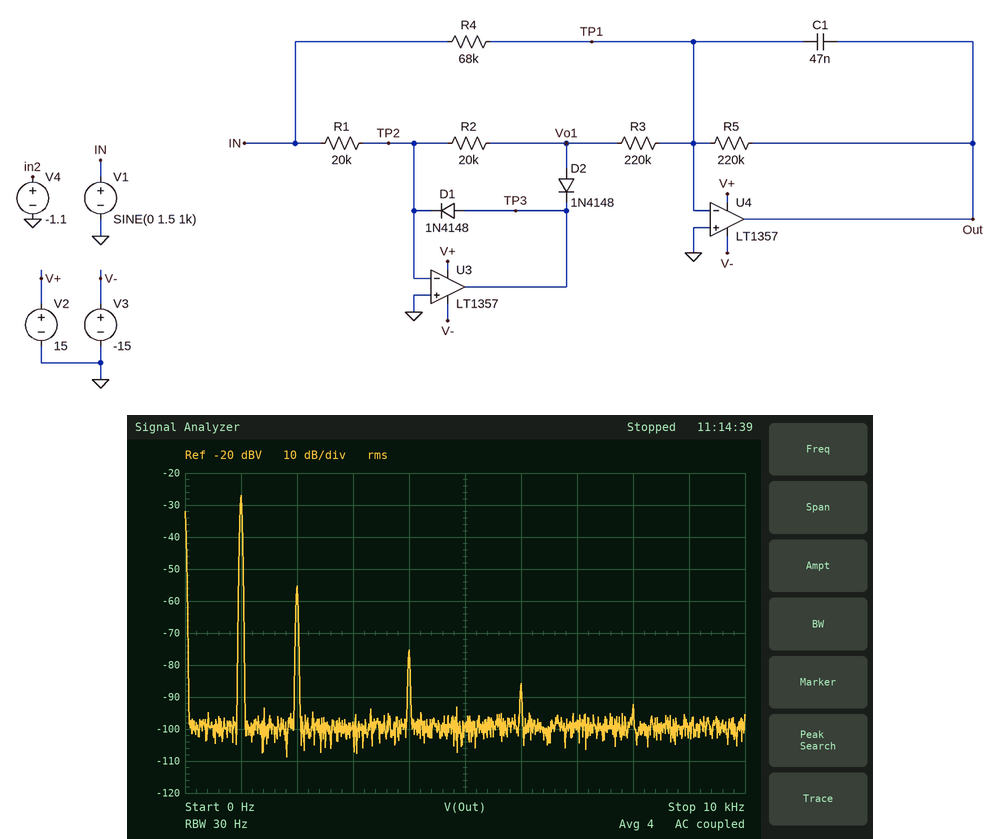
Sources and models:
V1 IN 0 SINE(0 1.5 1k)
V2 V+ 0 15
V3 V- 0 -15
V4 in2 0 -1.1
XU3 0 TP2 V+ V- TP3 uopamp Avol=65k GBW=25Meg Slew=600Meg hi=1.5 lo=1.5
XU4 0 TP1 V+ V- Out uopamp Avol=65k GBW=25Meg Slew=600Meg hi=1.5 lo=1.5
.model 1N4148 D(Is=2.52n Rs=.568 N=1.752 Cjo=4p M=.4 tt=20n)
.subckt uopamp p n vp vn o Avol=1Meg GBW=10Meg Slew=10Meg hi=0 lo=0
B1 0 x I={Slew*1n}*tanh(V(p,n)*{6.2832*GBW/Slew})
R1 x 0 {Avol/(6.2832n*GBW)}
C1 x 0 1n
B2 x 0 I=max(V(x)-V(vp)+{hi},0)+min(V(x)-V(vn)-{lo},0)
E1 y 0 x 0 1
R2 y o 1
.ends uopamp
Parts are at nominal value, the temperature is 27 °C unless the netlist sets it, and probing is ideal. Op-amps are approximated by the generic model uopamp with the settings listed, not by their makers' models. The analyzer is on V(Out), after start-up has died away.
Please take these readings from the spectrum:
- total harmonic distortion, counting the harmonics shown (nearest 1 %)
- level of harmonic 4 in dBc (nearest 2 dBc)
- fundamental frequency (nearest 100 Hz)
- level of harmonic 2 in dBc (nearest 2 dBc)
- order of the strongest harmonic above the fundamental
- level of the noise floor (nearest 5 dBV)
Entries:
4 %
-48 dBc
1.0 kHz
-28 dBc
2
-100 dBV
